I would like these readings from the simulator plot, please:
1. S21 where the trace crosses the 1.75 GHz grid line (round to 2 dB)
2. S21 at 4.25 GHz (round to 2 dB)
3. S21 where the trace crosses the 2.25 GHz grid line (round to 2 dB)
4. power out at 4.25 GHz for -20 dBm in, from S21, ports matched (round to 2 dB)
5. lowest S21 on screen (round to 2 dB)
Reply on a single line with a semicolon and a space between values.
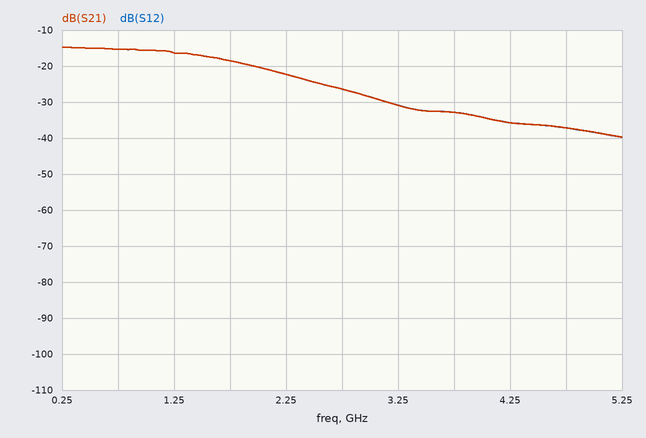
-18 dB; -36 dB; -22 dB; -56 dBm; -40 dB
